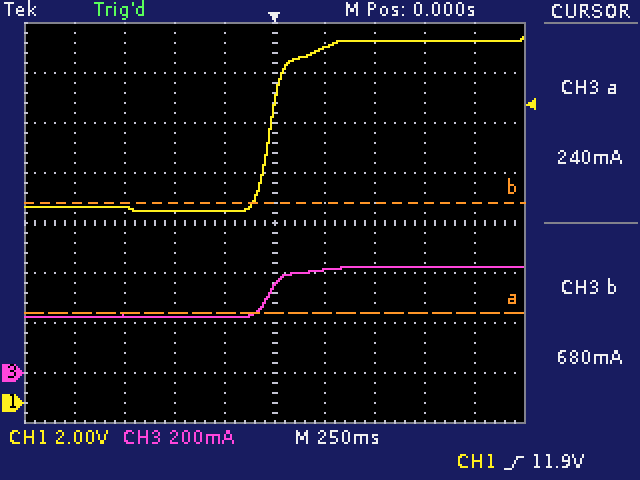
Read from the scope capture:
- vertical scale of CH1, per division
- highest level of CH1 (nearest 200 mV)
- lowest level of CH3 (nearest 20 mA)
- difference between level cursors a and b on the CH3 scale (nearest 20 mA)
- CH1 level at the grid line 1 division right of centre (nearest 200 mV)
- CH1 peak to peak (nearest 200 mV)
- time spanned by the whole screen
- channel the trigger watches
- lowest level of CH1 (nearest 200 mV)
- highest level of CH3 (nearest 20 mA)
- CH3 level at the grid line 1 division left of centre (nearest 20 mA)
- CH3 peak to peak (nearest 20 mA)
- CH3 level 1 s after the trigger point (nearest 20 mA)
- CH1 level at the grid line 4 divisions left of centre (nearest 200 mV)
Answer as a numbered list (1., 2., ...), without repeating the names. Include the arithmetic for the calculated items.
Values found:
1. 2 V
2. 14.6 V
3. 220 mA
4. 440 mA
5. 14.2 V
6. 14.6 V − (7.6 V) = 7.0 V
7. 2.5 s
8. CH1
9. 7.6 V
10. 420 mA
11. 220 mA
12. 420 mA − (220 mA) = 200 mA
13. 420 mA
14. 7.8 V
